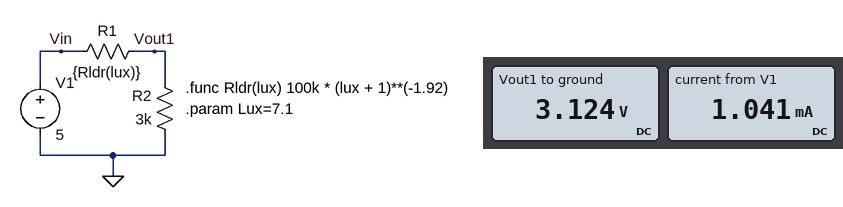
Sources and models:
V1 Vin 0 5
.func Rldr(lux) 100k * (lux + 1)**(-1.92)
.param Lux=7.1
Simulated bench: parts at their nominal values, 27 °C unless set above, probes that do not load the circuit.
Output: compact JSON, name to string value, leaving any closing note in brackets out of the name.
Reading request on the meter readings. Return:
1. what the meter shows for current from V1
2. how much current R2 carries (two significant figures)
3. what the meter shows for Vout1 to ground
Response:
{"what the meter shows for current from V1": "1.041 mA", "how much current R2 carries": "1.0 mA", "what the meter shows for Vout1 to ground": "3.124 V"}
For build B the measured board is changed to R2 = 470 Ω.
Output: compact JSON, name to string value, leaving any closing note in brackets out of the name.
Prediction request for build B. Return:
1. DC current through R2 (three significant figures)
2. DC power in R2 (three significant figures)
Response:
{"DC current through R2": "2.20 mA", "DC power in R2": "2.28 mW"}
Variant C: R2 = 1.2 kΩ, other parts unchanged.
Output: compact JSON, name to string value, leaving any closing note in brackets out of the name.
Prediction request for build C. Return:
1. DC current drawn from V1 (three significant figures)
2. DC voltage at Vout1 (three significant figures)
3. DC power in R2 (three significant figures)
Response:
{"DC current drawn from V1": "1.67 mA", "DC voltage at Vout1": "2.00 V", "DC power in R2": "3.33 mW"}
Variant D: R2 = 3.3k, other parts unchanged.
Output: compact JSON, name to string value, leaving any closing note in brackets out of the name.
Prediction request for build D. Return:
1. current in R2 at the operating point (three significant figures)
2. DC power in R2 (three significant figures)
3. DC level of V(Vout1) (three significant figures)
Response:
{"current in R2 at the operating point": "980 µA", "DC power in R2": "3.17 mW", "DC level of V(Vout1)": "3.23 V"}
